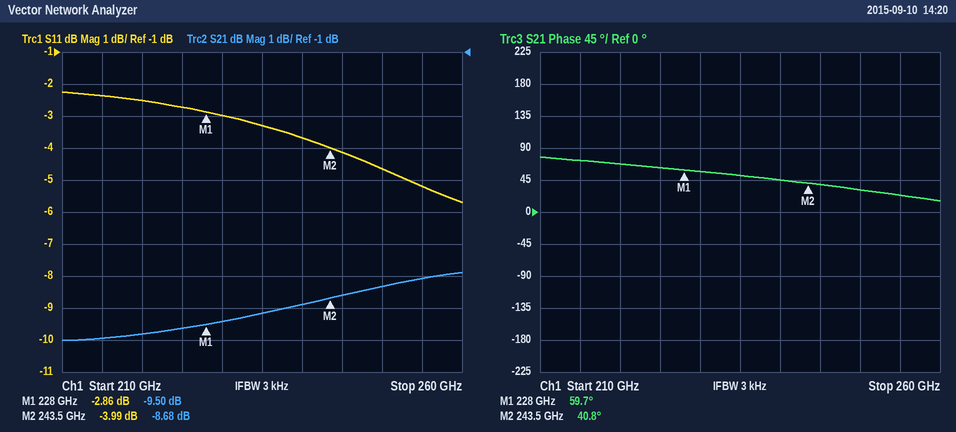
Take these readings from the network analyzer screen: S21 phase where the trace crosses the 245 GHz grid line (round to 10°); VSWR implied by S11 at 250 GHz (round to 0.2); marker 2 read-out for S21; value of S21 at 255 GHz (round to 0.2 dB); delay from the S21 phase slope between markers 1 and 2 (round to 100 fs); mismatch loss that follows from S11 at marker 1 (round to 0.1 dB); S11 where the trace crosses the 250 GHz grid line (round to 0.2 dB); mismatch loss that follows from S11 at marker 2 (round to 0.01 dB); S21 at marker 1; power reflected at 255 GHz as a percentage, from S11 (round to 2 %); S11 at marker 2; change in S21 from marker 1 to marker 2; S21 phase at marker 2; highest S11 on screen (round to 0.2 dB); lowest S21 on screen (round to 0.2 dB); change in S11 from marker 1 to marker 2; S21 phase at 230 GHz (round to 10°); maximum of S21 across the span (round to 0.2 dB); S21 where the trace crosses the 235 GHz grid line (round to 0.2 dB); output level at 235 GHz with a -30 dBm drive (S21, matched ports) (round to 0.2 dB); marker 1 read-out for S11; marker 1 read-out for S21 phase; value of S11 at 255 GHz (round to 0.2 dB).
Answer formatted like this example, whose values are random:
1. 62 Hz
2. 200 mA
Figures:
1. 40°
2. 3.8
3. -8.68 dB
4. -8.0 dB
5. 3.4 ps
6. 3.2 dB
7. -4.6 dB
8. 2.21 dB
9. -9.50 dB
10. 30 %
11. -3.99 dB
12. 0.82 dB
13. 40.8°
14. -2.2 dB
15. -10.0 dB
16. -1.13 dB
17. 60°
18. -7.8 dB
19. -9.2 dB
20. -39.2 dBm
21. -2.86 dB
22. 59.7°
23. -5.2 dB
